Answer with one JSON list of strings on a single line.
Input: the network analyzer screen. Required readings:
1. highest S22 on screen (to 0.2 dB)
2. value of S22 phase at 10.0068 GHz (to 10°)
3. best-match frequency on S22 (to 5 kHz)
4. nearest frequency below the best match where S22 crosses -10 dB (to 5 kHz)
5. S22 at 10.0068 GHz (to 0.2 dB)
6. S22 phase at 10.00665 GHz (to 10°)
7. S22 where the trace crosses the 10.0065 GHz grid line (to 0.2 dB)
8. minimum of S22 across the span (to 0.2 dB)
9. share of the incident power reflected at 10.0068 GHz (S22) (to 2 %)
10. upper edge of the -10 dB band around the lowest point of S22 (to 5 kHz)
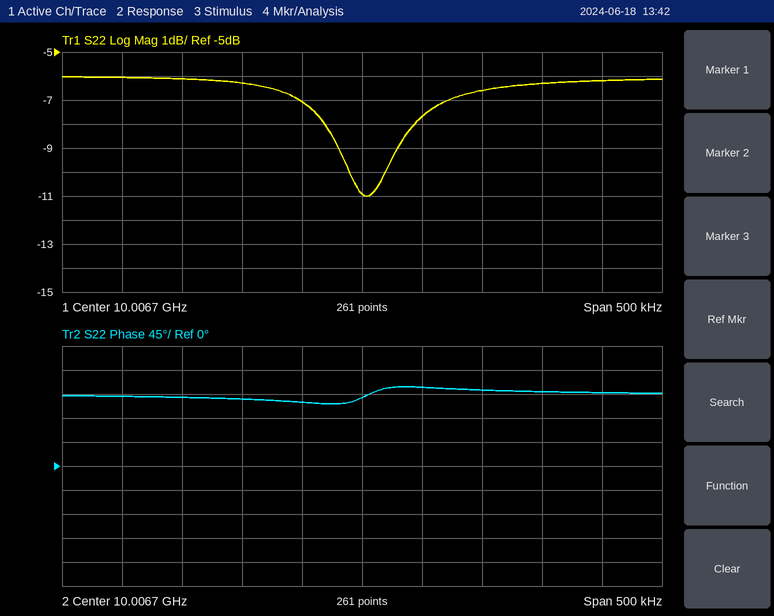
["-6.0 dB", "140°", "10.006705 GHz", "10.006690 GHz", "-6.6 dB", "120°", "-6.0 dB", "-11.0 dB", "22 %", "10.006720 GHz"]
